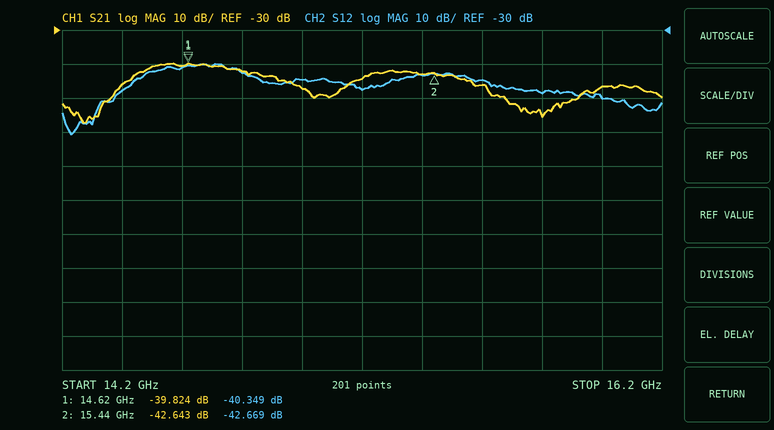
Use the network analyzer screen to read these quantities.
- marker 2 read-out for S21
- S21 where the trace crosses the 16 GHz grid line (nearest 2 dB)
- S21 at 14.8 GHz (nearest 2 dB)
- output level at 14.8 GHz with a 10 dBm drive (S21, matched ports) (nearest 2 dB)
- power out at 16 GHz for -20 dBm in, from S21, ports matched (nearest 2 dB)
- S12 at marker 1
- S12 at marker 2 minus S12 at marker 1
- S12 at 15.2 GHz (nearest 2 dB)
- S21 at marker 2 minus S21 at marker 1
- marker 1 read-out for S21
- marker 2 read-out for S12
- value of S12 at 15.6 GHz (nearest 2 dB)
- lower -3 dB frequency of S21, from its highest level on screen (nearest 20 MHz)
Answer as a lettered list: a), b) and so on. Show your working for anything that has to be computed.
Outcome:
a) -42.643 dB
b) -46 dB
c) -42 dB
d) 10 dBm + (-42 dB) = -32 dBm
e) -20 dBm + (-46 dB) = -66 dBm
f) -40.349 dB
g) -42.669 − (-40.349) = -2.320 dB
h) -48 dB
i) -42.643 − (-39.824) = -2.819 dB
j) -39.824 dB
k) -42.669 dB
l) -44 dB
m) 14.44 GHz
